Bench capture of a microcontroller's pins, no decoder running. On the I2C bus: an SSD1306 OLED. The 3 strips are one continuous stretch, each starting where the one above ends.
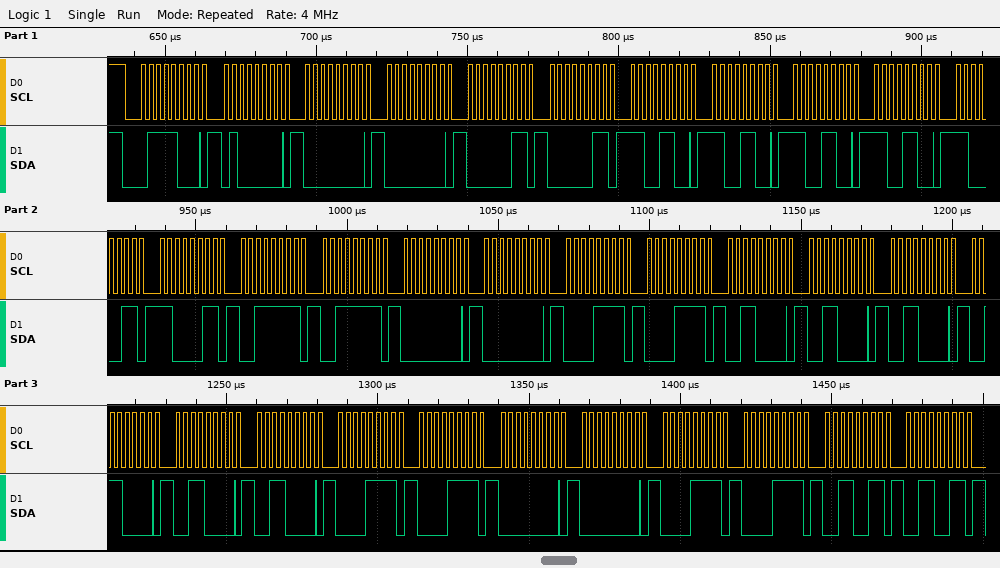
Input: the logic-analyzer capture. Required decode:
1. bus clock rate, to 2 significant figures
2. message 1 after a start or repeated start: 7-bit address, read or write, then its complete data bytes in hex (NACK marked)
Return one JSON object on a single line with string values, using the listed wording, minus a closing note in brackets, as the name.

{"bus clock rate, to 2 significant figures": "400 kHz", "message 1 after a start or repeated start: 7-bit address, read or write, then its complete data bytes in hex": "0x3C write: 40 00 00 03 03 CC CC CC CC C3 C3 3F 3F 00 00 0F 0F 30 30 30 30 30 30 0F 0F 00 00 0F 0F 33 33"}
